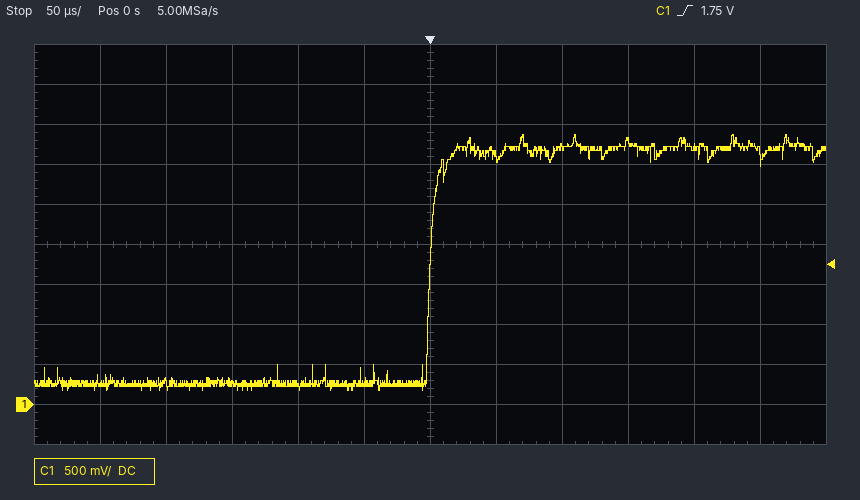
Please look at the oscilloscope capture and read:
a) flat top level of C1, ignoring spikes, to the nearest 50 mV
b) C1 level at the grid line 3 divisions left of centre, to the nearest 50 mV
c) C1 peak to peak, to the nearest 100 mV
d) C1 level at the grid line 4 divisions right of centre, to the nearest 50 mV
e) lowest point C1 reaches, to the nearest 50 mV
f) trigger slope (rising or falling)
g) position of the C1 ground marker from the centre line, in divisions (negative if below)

3.20 V
250 mV
3.20 V
3.20 V
200 mV
rising
-4.0 div
